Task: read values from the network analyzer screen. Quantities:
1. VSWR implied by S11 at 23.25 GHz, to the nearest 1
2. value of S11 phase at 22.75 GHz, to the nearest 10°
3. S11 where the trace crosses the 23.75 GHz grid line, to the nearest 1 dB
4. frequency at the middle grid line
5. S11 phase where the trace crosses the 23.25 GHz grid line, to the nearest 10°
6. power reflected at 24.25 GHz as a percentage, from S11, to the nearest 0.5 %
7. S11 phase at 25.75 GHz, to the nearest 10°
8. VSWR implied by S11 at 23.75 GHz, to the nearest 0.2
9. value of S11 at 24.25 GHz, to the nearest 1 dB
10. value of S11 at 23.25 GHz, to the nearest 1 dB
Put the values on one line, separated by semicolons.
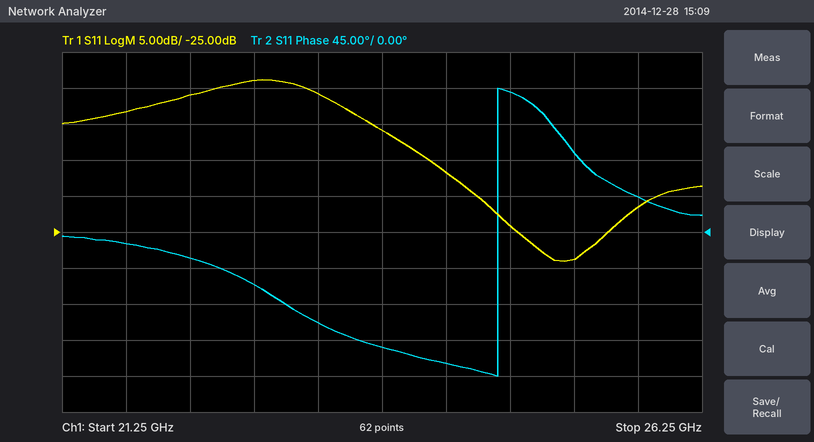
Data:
3; -70°; -11 dB; 23.75 GHz; -110°; 2.0 %; 40°; 1.8; -17 dB; -6 dB
